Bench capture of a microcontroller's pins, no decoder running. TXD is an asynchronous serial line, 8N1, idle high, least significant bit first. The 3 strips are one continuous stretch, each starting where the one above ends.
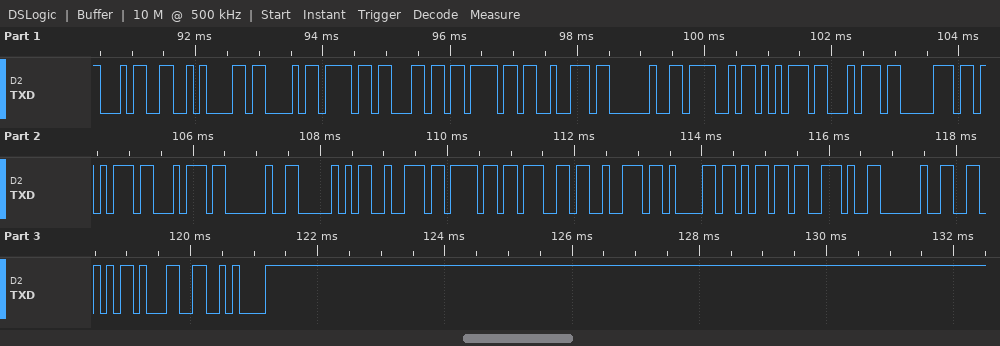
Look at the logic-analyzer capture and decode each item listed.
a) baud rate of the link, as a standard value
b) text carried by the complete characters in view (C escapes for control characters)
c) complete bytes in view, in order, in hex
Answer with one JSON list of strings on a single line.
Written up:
["9600 baud", "\"4\\nColor Output Program. V1\\n\"", "0x34 0x0A 0x43 0x6F 0x6C 0x6F 0x72 0x20 0x4F 0x75 0x74 0x70 0x75 0x74 0x20 0x50 0x72 0x6F 0x67 0x72 0x61 0x6D 0x2E 0x20 0x56 0x31 0x0A"]
